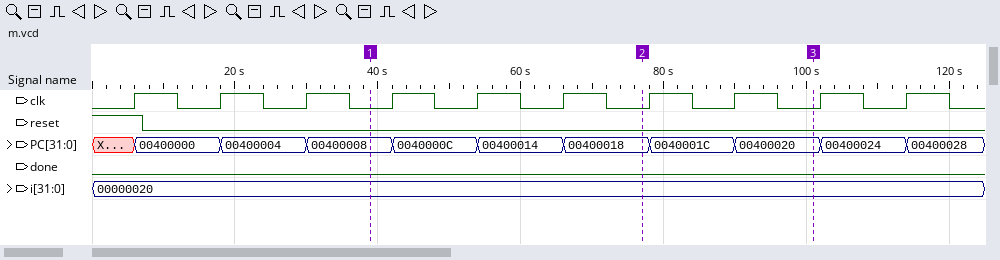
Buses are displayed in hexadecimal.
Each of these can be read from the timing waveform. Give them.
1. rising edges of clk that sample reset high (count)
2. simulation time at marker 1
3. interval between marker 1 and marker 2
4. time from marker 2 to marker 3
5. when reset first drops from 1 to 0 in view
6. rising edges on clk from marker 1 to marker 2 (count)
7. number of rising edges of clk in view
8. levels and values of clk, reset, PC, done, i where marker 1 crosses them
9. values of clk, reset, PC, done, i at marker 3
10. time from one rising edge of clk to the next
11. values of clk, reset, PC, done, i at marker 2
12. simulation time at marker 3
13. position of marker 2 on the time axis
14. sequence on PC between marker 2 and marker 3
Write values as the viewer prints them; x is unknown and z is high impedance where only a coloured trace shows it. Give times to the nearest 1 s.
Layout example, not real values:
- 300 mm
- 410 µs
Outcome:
- 1
- 39 s
- 38 s
- 24 s
- 7 s
- 3
- 10
- clk=0, reset=0, PC=00400008, done=0, i=00000020
- clk=0, reset=0, PC=00400020, done=0, i=00000020
- 12 s
- clk=0, reset=0, PC=00400018, done=0, i=00000020
- 101 s
- 77 s
- 00400018, 0040001C, 00400020
